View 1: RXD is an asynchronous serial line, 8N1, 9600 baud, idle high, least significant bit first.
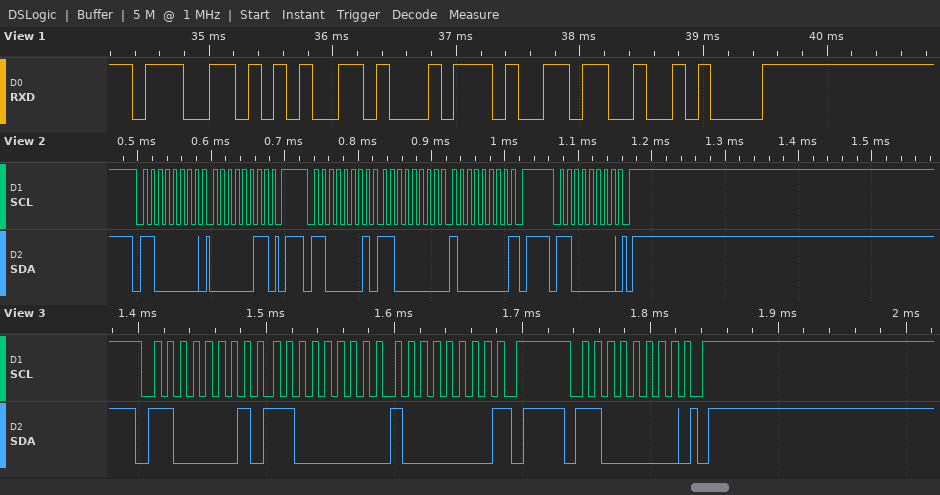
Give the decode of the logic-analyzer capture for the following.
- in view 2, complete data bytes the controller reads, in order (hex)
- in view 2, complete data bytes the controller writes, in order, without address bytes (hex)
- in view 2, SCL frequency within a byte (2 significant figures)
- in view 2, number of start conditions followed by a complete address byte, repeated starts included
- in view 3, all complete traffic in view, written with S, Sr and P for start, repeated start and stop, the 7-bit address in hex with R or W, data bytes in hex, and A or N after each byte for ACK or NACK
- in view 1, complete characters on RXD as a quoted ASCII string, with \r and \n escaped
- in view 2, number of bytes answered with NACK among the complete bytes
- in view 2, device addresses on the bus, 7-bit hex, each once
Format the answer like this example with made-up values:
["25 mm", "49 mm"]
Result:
["C0 80", "03", "100 kHz", "3", "S 60R A C0 A 80 N P S 60W A P", "\"get6\\n\"", "1", "0x60"]
